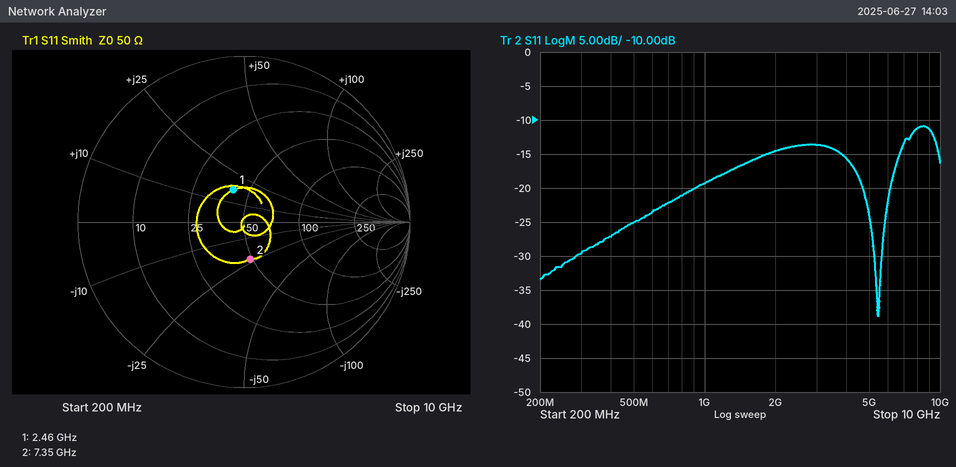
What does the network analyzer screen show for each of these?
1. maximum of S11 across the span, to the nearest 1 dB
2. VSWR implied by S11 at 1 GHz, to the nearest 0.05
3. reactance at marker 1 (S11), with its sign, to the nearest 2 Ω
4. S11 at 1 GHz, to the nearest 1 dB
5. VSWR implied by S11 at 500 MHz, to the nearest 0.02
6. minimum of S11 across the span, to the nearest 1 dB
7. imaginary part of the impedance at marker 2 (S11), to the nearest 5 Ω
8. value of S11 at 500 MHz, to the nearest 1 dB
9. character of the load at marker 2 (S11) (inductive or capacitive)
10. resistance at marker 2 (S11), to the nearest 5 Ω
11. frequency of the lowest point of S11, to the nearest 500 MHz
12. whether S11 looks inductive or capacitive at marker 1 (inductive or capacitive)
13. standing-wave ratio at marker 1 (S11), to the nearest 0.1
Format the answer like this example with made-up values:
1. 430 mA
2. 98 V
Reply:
1. -11 dB
2. 1.25
3. +16 Ω
4. -19 dB
5. 1.12
6. -39 dB
7. -25 Ω
8. -25 dB
9. capacitive
10. 50 Ω
11. 5.5 GHz
12. inductive
13. 1.5
